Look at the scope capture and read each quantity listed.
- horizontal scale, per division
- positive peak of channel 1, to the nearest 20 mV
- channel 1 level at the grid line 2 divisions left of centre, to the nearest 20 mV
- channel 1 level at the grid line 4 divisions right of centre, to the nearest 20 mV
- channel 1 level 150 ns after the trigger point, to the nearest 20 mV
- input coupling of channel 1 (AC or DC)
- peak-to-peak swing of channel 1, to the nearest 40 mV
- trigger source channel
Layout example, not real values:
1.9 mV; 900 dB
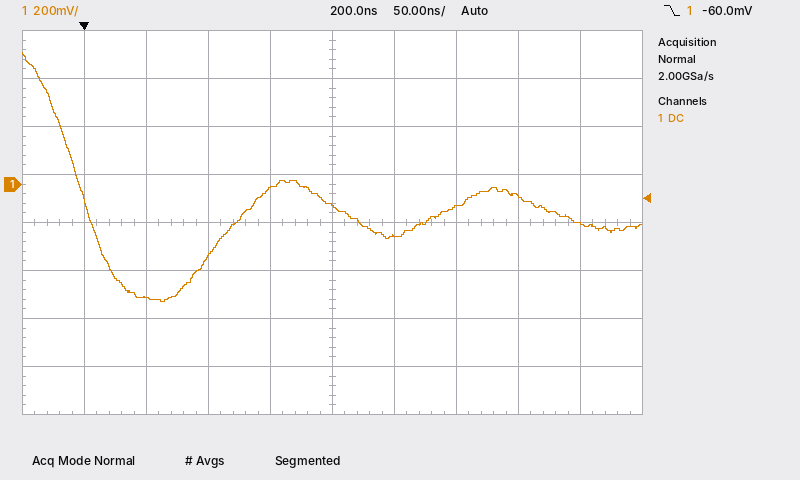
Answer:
50 ns; 540 mV; -300 mV; -160 mV; -20 mV; DC; 1.04 V; channel 1
